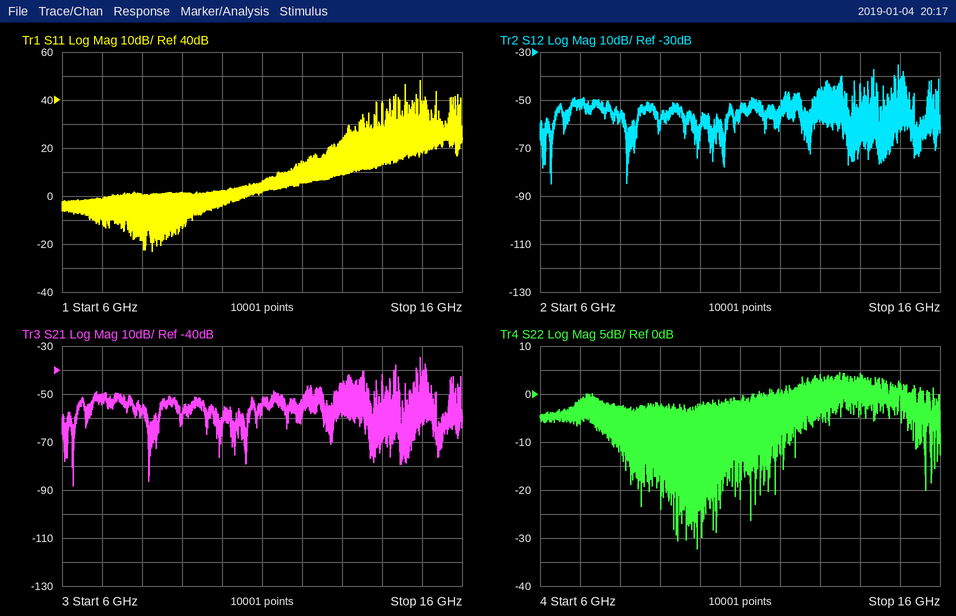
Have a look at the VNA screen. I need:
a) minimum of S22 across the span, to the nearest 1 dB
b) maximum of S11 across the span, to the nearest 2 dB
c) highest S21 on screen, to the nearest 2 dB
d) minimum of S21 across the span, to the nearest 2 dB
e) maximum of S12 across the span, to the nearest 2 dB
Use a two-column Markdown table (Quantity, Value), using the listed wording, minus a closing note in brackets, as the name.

| Quantity | Value |
|---|---|
| minimum of S22 across the span, to the nearest 1 dB | -32 dB |
| maximum of S11 across the span, to the nearest 2 dB | 48 dB |
| highest S21 on screen, to the nearest 2 dB | -34 dB |
| minimum of S21 across the span, to the nearest 2 dB | -88 dB |
| maximum of S12 across the span, to the nearest 2 dB | -36 dB |
